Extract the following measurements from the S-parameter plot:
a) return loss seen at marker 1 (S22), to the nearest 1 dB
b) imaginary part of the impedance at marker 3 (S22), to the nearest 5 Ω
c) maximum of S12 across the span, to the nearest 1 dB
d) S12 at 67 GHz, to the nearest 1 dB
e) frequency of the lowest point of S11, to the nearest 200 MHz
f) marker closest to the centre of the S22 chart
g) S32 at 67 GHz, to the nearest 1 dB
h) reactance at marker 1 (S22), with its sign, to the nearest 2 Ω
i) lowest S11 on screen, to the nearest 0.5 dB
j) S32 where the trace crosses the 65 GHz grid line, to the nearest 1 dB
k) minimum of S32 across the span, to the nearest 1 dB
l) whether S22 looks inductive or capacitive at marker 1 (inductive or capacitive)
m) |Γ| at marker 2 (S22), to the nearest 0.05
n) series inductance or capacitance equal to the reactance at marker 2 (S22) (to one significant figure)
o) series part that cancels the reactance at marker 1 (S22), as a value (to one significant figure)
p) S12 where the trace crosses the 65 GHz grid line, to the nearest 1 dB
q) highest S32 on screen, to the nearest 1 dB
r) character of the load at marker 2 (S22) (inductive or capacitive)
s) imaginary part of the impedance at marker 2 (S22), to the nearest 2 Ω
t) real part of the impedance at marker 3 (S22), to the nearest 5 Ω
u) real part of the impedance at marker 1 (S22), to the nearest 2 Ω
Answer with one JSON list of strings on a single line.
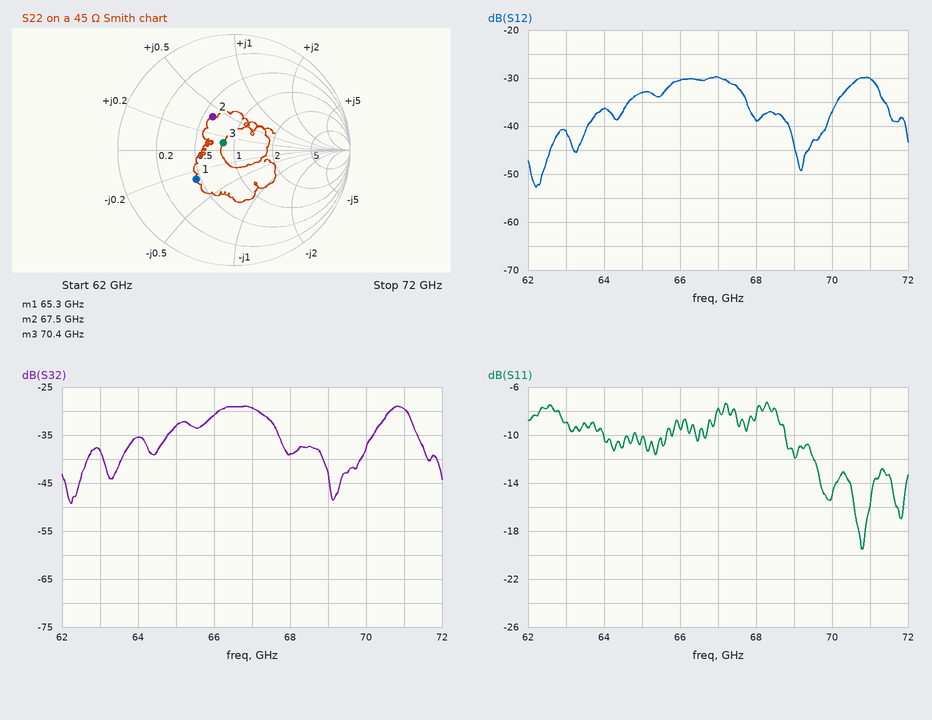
["8 dB", "+5 Ω", "-30 dB", "-30 dB", "70.8 GHz", "marker 3", "-29 dB", "-12 Ω", "-19.5 dB", "-33 dB", "-49 dB", "capacitive", "0.35", "40 pH", "30 pH", "-33 dB", "-29 dB", "inductive", "+18 Ω", "35 Ω", "20 Ω"]
